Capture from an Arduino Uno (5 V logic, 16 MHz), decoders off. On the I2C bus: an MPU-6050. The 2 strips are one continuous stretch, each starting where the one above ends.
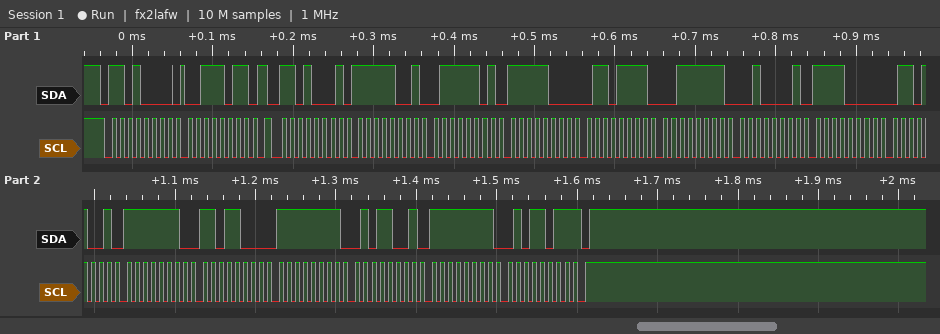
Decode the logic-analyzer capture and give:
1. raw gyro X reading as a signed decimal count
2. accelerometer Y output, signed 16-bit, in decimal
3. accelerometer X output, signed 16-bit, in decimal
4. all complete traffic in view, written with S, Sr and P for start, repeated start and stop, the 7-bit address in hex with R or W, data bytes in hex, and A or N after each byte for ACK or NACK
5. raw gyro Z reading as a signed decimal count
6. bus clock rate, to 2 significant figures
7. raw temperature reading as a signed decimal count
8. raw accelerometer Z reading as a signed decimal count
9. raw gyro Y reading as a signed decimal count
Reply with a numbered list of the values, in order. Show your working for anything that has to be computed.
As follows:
1. 0xFED8 = -296
2. 0xF86F = -1937
3. 0xF97D = -1667
4. S 68W A 3B A Sr 68R A F9 A 7D A F8 A 6F A 3F A 21 A F0 A 69 A FE A D8 A FF A 59 A FF A 5B N P
5. 0xFF5B = -165
6. 100 kHz
7. 0xF069 = -3991
8. 0x3F21 = 16161
9. 0xFF59 = -167
